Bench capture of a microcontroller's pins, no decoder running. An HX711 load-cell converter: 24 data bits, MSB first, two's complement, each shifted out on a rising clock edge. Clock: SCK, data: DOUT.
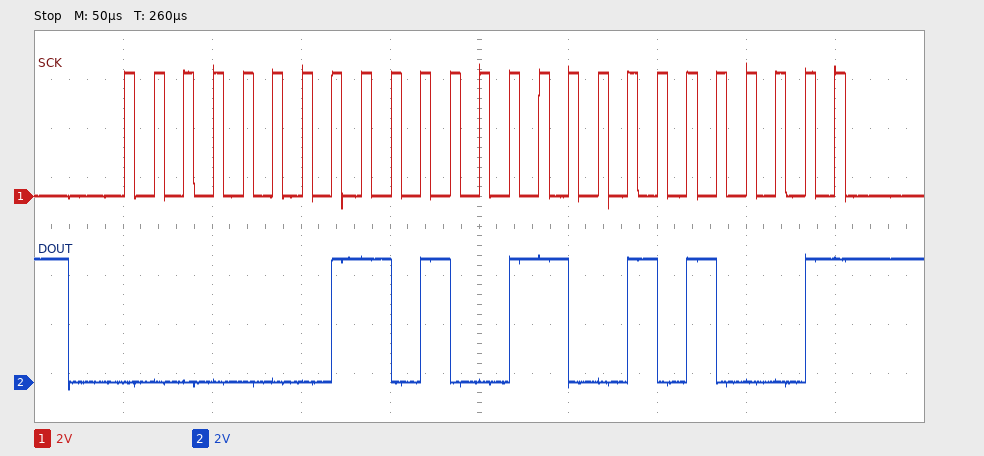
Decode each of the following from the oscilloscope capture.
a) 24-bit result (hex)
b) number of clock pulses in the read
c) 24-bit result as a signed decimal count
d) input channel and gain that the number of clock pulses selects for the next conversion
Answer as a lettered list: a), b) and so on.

a) 0x01A651
b) 25
c) 108113
d) channel A, gain 128
